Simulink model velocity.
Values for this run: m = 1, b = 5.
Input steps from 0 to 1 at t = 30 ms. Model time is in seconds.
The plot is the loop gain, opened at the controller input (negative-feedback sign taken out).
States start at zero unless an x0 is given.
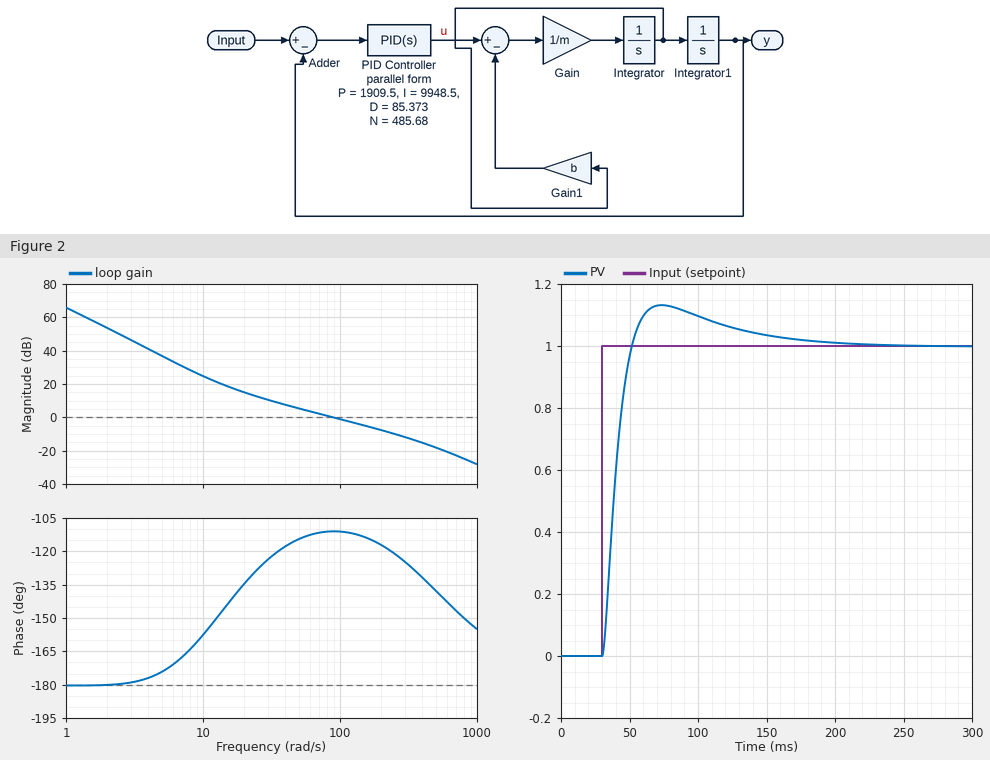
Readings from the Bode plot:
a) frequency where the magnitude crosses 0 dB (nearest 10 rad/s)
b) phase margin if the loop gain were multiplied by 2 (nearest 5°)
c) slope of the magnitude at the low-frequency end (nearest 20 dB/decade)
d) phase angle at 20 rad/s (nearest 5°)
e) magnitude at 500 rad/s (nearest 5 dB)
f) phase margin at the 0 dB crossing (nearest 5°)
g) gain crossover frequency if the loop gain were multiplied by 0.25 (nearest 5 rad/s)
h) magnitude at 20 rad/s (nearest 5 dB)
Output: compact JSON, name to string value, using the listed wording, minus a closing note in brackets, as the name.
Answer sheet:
{"frequency where the magnitude crosses 0 dB": "90 rad/s", "phase margin if the loop gain were multiplied by 2": "65°", "slope of the magnitude at the low-frequency end": "-40 dB/decade", "phase angle at 20 rad/s": "-135°", "magnitude at 500 rad/s": "-20 dB", "phase margin at the 0 dB crossing": "70°", "gain crossover frequency if the loop gain were multiplied by 0.25": "25 rad/s", "magnitude at 20 rad/s": "15 dB"}
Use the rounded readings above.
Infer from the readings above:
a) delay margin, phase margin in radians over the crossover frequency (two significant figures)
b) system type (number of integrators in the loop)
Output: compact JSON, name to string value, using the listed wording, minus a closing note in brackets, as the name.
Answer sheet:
{"delay margin, phase margin in radians over the crossover frequency": "0.014 s", "system type": "2"}
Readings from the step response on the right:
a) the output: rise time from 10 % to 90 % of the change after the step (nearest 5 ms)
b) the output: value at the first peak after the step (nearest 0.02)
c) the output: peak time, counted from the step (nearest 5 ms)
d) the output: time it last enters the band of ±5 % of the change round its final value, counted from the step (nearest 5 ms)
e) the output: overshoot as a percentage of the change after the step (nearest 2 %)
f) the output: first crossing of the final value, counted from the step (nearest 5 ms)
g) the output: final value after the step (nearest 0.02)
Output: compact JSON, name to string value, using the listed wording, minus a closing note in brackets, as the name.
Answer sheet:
{"the output: rise time from 10 % to 90 % of the change after the step": "15 ms", "the output: value at the first peak after the step": "1.14", "the output: peak time, counted from the step": "45 ms", "the output: time it last enters the band of ±5 % of the change round its final value, counted from the step": "105 ms", "the output: overshoot as a percentage of the change after the step": "14 %", "the output: first crossing of the final value, counted from the step": "20 ms", "the output: final value after the step": "1.00"}
